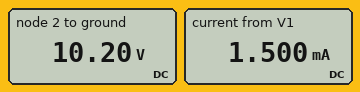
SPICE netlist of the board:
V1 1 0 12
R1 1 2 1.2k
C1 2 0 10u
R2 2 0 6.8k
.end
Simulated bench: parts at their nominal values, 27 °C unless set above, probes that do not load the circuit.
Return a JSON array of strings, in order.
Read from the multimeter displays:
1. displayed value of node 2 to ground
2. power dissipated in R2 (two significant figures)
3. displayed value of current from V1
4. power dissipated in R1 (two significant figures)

["10.20 V", "15 mW", "1.500 mA", "2.7 mW"]
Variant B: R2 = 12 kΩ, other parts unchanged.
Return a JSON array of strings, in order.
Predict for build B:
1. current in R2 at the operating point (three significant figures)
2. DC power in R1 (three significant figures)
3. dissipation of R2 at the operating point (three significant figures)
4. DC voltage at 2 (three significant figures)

["909 µA", "992 µW", "9.92 mW", "10.9 V"]
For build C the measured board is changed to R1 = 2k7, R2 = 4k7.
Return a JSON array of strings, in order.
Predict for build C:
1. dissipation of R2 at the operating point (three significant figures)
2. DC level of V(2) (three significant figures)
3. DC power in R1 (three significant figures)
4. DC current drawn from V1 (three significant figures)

["12.4 mW", "7.62 V", "7.10 mW", "1.62 mA"]
